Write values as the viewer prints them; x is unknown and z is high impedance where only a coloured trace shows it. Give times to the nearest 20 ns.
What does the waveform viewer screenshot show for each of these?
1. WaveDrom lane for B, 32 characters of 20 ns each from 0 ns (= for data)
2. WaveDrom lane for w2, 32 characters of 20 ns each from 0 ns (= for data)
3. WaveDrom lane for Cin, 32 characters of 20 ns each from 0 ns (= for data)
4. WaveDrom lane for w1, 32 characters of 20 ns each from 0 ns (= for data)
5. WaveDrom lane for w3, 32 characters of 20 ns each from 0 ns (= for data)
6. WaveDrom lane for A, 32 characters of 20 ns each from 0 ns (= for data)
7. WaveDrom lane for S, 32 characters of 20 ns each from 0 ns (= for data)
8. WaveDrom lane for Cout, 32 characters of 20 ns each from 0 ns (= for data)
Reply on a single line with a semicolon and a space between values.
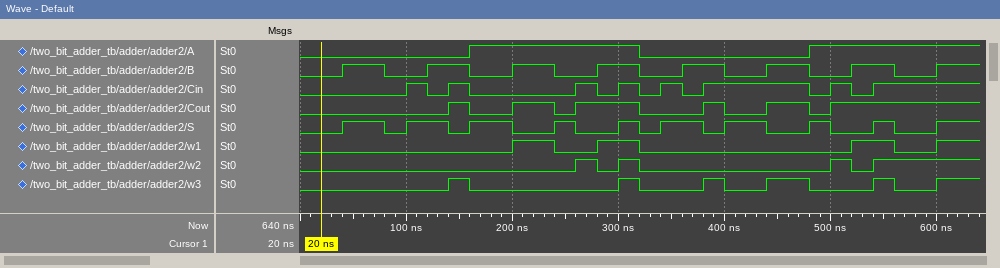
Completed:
{name: 'B', wave: '0.1.0.1.0.1.0.1.0.1.0.1.0.1.0.1.'}; {name: 'w2', wave: '0............1010........101....'}; {name: 'Cin', wave: '0....1010....1010101....0101....'}; {name: 'w1', wave: '0.........1.0.1.0.........1.0.1.'}; {name: 'w3', wave: '0......10......10..10.1.0..10.1.'}; {name: 'A', wave: '0.......1.......0.......1.......'}; {name: 'S', wave: '0.1.01.01.0.10.101.01.0.10.10.1.'}; {name: 'Cout', wave: '0......10.1.01..0..10.1.01......'}
